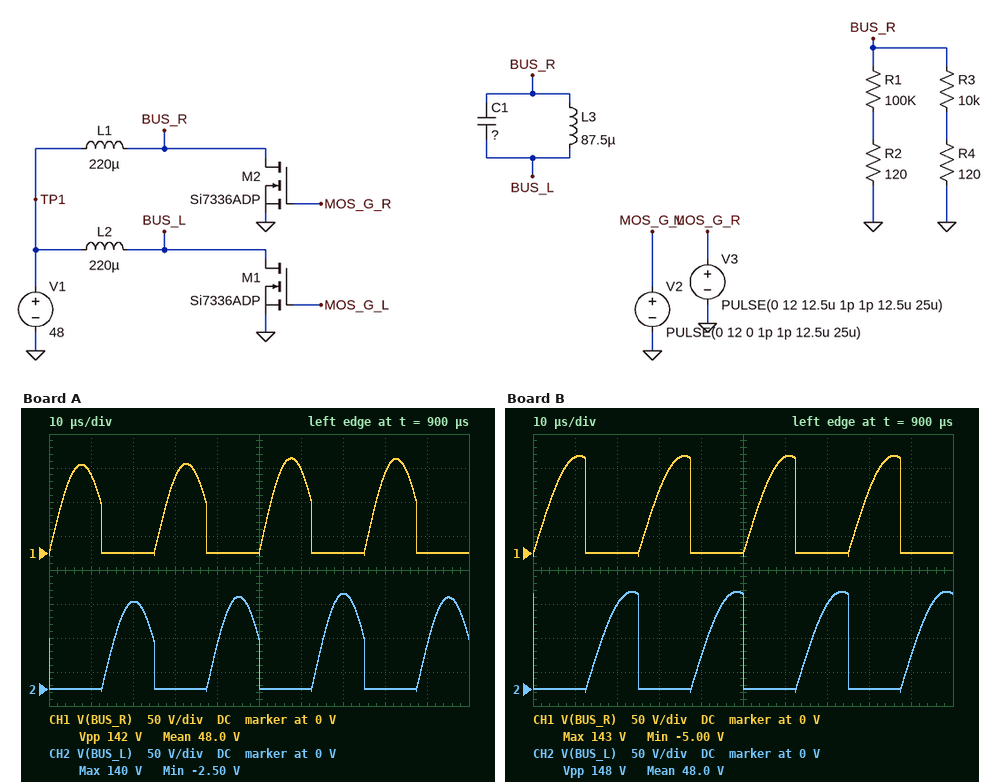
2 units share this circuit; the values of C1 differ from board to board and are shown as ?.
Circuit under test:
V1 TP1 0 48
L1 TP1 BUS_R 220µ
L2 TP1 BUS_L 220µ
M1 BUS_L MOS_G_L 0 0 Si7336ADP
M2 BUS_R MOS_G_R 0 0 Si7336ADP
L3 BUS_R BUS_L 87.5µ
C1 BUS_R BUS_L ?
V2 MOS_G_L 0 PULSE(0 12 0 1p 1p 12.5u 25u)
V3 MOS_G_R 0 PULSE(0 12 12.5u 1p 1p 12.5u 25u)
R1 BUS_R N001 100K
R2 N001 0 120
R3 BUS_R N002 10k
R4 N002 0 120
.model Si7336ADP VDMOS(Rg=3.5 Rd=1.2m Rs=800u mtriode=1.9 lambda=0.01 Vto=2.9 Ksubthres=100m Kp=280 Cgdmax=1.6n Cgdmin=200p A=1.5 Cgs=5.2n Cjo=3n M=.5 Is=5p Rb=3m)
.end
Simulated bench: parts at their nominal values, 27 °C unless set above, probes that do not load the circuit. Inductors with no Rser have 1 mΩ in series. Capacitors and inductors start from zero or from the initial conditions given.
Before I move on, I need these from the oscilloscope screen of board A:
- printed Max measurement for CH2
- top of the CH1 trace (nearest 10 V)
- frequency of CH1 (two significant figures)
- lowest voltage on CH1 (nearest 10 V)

140 V
140 V
40 kHz
0 V
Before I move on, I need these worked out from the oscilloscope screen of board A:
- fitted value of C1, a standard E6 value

330 nF
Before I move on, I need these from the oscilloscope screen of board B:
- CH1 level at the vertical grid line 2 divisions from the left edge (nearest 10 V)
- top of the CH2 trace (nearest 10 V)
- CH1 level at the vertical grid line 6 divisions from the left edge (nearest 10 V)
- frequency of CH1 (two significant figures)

0 V
140 V
140 V
40 kHz
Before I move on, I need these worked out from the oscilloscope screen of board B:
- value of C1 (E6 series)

680 nF
